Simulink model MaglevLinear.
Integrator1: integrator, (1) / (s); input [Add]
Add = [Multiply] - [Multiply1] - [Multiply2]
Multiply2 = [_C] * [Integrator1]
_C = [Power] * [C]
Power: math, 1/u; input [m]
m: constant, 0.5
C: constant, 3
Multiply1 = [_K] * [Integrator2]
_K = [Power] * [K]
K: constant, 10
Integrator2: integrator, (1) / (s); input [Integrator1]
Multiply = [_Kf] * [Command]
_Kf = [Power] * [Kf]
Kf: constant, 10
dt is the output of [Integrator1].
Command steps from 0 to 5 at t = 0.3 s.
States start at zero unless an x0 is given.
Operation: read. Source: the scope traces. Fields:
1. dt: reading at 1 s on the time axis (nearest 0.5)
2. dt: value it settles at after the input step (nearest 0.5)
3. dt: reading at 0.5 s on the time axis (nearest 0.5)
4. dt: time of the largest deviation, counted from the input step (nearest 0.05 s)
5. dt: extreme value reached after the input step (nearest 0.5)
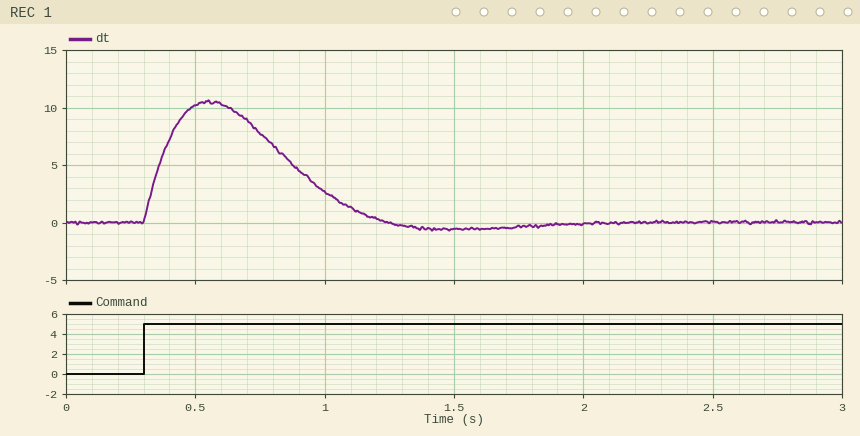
2.5
0.0
10.0
0.25 s
10.5
